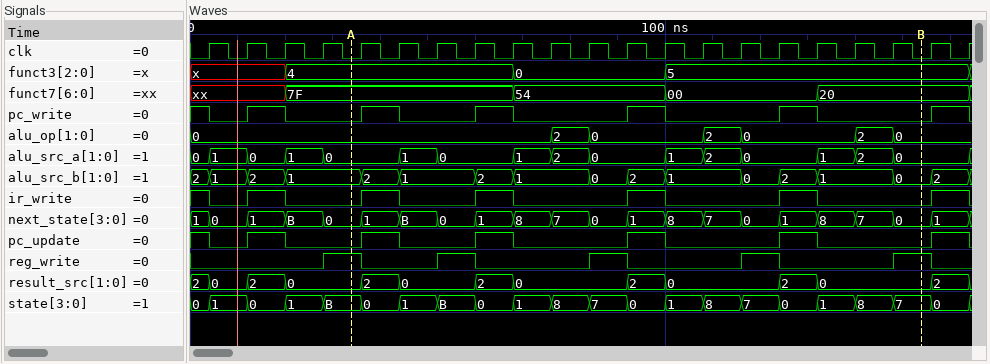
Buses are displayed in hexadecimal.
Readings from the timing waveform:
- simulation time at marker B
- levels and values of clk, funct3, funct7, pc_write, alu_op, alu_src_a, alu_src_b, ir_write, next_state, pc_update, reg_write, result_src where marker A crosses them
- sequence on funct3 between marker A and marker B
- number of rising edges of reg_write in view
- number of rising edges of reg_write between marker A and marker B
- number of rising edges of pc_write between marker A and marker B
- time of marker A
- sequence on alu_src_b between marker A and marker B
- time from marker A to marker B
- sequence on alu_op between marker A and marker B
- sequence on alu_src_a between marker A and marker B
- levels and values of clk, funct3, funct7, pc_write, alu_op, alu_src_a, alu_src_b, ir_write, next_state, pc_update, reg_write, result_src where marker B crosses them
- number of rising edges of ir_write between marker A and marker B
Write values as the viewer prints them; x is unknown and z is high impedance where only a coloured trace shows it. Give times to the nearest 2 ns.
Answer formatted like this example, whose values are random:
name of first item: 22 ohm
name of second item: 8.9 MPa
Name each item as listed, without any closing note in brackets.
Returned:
simulation time at marker B: 154 ns
levels and values of clk, funct3, funct7, pc_write, alu_op, alu_src_a, alu_src_b, ir_write, next_state, pc_update, reg_write, result_src where marker A crosses them: clk=0, funct3=4, funct7=7F, pc_write=0, alu_op=0, alu_src_a=0, alu_src_b=1, ir_write=0, next_state=0, pc_update=0, reg_write=1, result_src=0
sequence on funct3 between marker A and marker B: 4, 0, 5
number of rising edges of reg_write in view: 5
number of rising edges of reg_write between marker A and marker B: 4
number of rising edges of pc_write between marker A and marker B: 4
time of marker A: 34 ns
sequence on alu_src_b between marker A and marker B: 1, 2, 1, 2, 1, 0, 2, 1, 0, 2, 1, 0
time from marker A to marker B: 120 ns
sequence on alu_op between marker A and marker B: 0, 2, 0, 2, 0, 2, 0
sequence on alu_src_a between marker A and marker B: 0, 1, 0, 1, 2, 0, 1, 2, 0, 1, 2, 0
levels and values of clk, funct3, funct7, pc_write, alu_op, alu_src_a, alu_src_b, ir_write, next_state, pc_update, reg_write, result_src where marker B crosses them: clk=0, funct3=5, funct7=20, pc_write=0, alu_op=0, alu_src_a=0, alu_src_b=0, ir_write=0, next_state=0, pc_update=0, reg_write=1, result_src=0
number of rising edges of ir_write between marker A and marker B: 4
